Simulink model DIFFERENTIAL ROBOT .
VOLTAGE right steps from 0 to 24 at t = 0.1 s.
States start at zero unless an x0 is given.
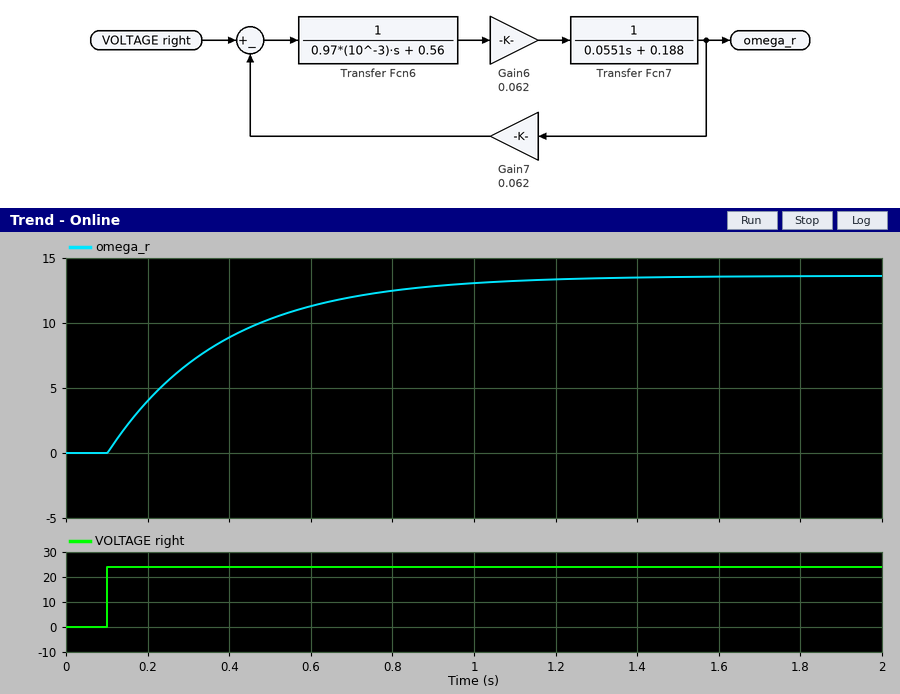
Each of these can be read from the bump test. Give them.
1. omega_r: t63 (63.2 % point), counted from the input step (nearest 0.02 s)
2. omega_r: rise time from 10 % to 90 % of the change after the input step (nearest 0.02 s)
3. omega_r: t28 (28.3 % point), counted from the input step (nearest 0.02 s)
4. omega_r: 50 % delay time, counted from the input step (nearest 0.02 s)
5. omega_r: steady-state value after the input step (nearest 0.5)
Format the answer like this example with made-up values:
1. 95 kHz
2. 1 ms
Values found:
1. 0.28 s
2. 0.62 s
3. 0.10 s
4. 0.20 s
5. 13.5
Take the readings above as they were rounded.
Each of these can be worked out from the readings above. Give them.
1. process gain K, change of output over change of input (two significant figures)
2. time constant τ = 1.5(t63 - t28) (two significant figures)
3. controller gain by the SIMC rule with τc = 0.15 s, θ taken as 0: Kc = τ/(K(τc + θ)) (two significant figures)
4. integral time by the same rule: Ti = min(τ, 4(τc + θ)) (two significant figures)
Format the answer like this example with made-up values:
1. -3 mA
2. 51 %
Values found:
1. 0.56
2. 0.27 s
3. 3.2
4. 0.27 s
